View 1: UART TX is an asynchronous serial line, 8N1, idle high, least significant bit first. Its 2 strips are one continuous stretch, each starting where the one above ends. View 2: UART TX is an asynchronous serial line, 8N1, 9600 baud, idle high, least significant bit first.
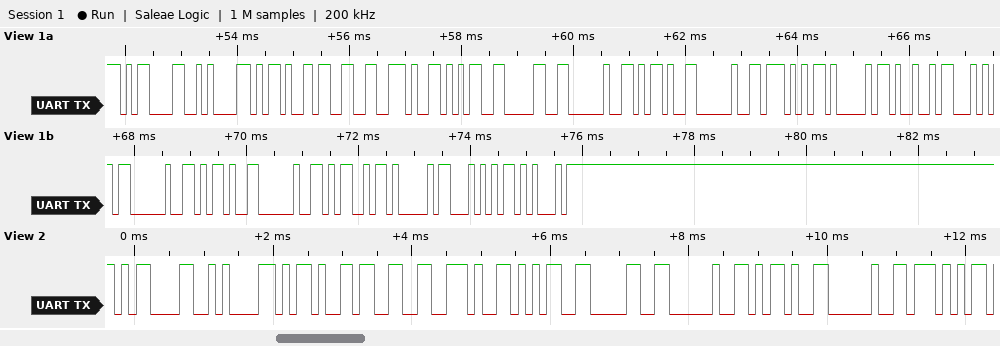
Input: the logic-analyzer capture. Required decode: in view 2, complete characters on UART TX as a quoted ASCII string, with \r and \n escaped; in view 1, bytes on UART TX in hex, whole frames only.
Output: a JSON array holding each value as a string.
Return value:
["\"\\r\\n-3.50 - W\"", "0x0D 0x0A 0x2D 0x33 0x2E 0x35 0x30 0x20 0x2D 0x20 0x57 0x41 0x49 0x54 0x20 0x2D 0x20 0x4D 0x41 0x54 0x45"]
